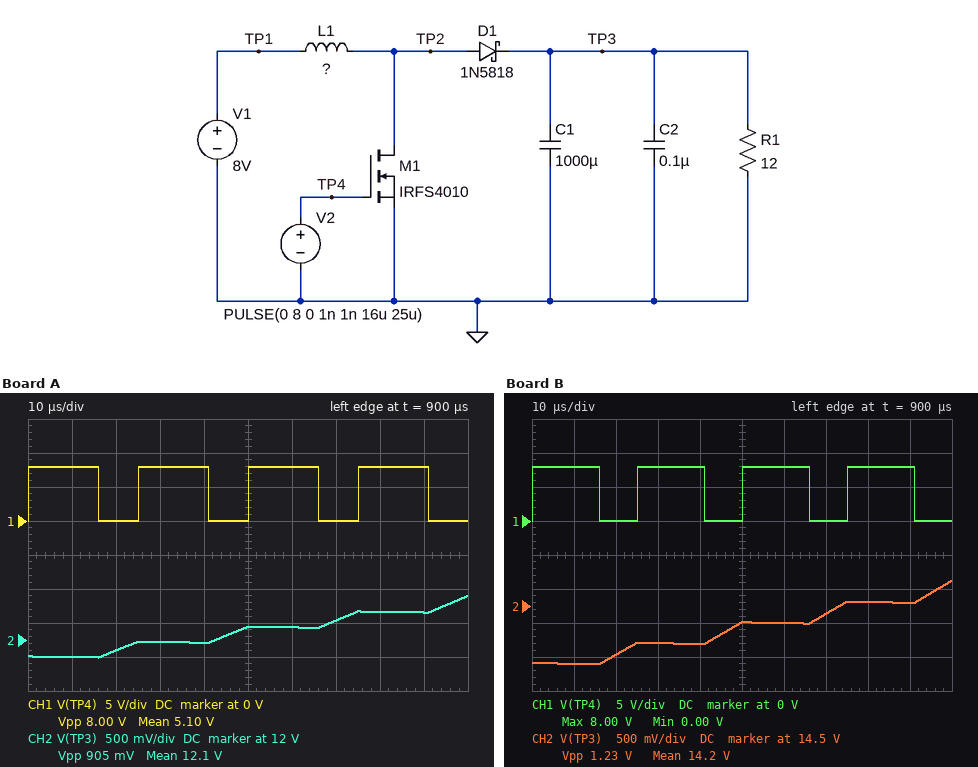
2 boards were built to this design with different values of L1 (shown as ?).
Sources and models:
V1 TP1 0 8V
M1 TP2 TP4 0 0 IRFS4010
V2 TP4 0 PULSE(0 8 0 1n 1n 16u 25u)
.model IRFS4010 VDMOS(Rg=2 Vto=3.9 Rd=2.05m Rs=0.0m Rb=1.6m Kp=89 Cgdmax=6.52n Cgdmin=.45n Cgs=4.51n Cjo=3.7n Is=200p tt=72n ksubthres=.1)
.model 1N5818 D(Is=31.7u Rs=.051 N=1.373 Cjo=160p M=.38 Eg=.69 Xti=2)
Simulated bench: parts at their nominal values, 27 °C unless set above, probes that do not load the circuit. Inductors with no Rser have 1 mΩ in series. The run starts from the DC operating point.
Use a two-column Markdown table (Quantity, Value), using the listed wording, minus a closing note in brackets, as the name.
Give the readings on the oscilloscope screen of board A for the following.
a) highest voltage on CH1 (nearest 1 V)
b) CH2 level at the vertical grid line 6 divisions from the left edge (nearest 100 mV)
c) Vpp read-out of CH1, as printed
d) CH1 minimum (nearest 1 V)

| Quantity | Value |
|---|---|
| highest voltage on CH1 | 8 V |
| CH2 level at the vertical grid line 6 divisions from the left edge | 12.2 V |
| Vpp read-out of CH1, as printed | 8.00 V |
| CH1 minimum | 0 V |
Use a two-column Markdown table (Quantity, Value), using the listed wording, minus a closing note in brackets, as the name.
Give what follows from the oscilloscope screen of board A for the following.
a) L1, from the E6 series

| Quantity | Value |
|---|---|
| L1, from the E6 series | 150 µH |
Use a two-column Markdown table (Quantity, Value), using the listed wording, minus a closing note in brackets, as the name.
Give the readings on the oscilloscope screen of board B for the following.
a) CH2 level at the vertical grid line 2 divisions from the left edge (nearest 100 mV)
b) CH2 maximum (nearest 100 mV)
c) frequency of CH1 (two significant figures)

| Quantity | Value |
|---|---|
| CH2 level at the vertical grid line 2 divisions from the left edge | 13.8 V |
| CH2 maximum | 14.9 V |
| frequency of CH1 | 40 kHz |
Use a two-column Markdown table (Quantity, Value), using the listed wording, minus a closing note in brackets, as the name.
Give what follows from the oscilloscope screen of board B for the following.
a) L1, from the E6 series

| Quantity | Value |
|---|---|
| L1, from the E6 series | 100 µH |
